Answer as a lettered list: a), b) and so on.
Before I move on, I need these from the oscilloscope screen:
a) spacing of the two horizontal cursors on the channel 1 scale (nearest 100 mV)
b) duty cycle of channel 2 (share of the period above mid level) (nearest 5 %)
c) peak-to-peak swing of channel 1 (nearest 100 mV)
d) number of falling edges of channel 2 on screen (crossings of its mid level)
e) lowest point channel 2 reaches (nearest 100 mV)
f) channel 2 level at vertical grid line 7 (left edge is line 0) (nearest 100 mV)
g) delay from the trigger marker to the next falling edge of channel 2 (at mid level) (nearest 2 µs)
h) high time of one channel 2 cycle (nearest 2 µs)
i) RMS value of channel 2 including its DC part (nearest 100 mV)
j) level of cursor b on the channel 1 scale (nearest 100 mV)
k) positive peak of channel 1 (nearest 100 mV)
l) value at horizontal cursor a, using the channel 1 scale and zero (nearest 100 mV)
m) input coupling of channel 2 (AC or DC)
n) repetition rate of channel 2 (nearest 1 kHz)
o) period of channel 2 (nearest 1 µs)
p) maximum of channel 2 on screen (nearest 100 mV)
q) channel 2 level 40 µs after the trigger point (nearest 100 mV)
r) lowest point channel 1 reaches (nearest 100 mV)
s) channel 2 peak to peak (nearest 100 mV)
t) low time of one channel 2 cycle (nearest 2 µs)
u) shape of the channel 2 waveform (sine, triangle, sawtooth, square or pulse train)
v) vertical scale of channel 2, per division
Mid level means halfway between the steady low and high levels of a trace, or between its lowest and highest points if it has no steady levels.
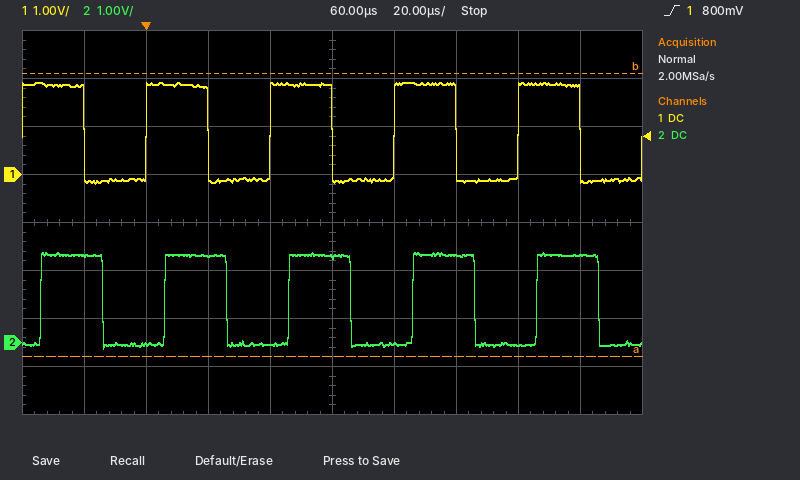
a) 5.9 V
b) 50 %
c) 2.1 V
d) 5
e) -100 mV
f) 1.8 V
g) 26 µs
h) 20 µs
i) 1.3 V
j) 2.1 V
k) 1.9 V
l) -3.8 V
m) DC
n) 25 kHz
o) 40 µs
p) 1.9 V
q) 0.0 V
r) -200 mV
s) 2.0 V
t) 20 µs
u) square
v) 1 V
